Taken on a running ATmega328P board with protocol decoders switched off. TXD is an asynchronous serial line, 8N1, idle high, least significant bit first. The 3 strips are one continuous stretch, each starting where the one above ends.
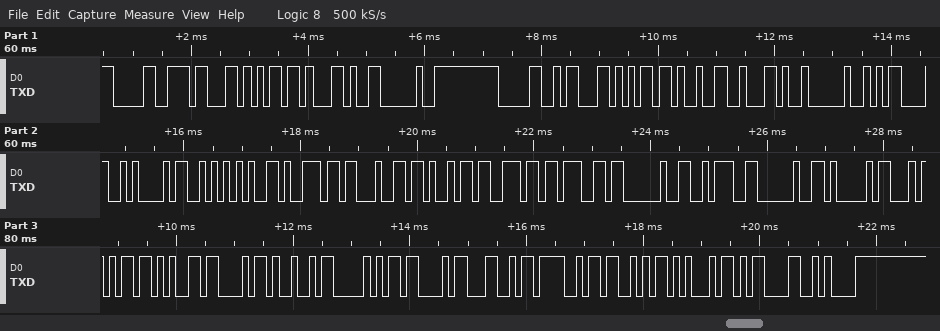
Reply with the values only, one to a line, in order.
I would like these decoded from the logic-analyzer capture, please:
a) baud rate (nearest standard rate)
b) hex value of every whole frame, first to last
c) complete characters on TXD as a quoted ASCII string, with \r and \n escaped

9600 baud
0x30 0x63 0x6D 0x2C 0x20 0x30 0x63 0x6D 0x32 0x2C 0x20 0x0D 0x0A 0x53 0x65 0x6E 0x64 0x69 0x6E 0x67 0x20 0x3A 0x20 0x41 0x54 0x2B 0x43 0x49 0x50 0x43 0x4C 0x4F 0x53 0x45 0x0D 0x0A
"0cm, 0cm2, \r\nSending : AT+CIPCLOSE\r\n"
